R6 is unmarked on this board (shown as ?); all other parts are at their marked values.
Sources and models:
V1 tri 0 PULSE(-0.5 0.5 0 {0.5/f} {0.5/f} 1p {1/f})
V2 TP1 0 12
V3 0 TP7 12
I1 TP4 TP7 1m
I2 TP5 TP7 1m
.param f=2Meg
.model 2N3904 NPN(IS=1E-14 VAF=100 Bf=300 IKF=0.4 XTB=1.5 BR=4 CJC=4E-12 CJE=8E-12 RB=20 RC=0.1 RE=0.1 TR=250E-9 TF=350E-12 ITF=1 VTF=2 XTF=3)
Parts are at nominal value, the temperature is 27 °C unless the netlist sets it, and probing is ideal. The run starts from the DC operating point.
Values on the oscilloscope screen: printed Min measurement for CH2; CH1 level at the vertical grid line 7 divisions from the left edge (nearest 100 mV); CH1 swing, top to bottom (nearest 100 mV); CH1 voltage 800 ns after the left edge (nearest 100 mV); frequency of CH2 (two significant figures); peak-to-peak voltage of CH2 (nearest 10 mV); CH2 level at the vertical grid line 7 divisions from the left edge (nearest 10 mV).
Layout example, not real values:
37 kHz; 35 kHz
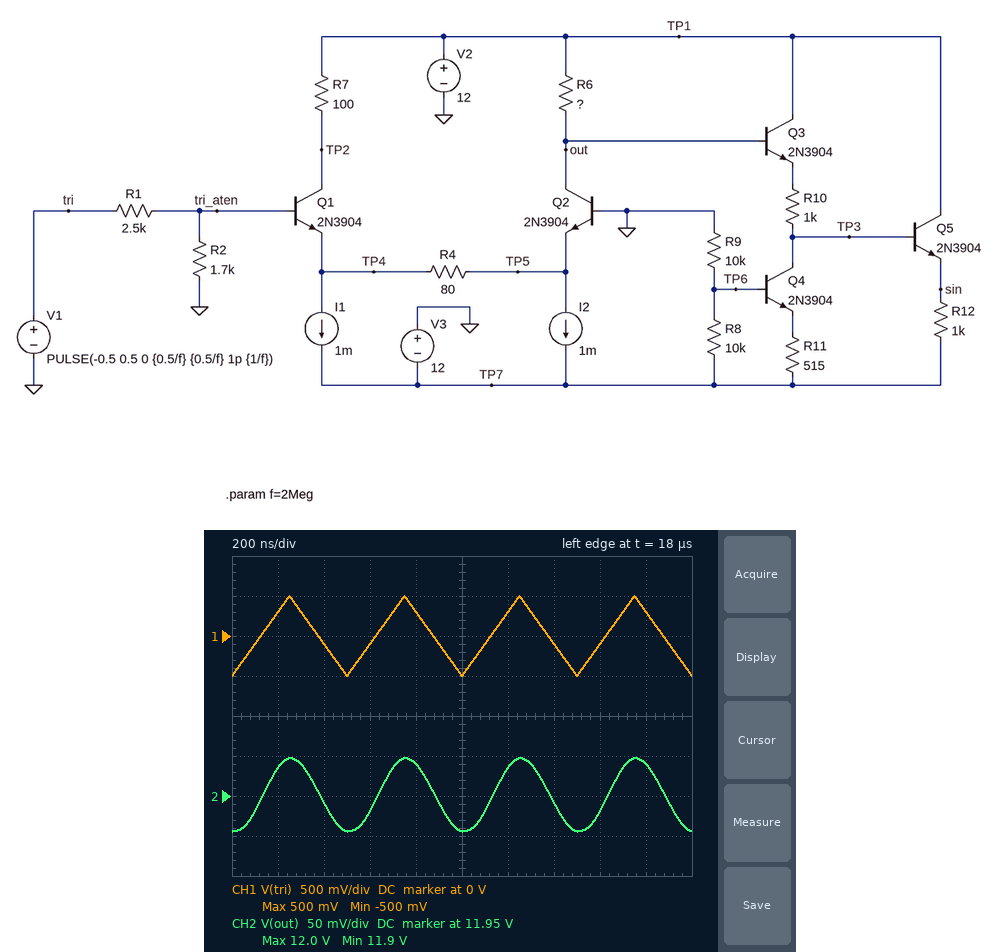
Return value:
11.9 V; -100 mV; 1.0 V; 300 mV; 2.0 MHz; 90 mV; 11.94 V
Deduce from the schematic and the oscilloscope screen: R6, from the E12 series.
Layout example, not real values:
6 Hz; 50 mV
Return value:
47 Ω
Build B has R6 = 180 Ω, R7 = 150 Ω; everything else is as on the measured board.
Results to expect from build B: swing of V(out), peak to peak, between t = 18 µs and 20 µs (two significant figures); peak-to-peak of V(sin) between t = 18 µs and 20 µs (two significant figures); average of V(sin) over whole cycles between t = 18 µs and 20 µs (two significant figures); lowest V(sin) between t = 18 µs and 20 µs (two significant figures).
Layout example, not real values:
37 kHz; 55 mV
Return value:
350 mV; 320 mV; 410 mV; 250 mV
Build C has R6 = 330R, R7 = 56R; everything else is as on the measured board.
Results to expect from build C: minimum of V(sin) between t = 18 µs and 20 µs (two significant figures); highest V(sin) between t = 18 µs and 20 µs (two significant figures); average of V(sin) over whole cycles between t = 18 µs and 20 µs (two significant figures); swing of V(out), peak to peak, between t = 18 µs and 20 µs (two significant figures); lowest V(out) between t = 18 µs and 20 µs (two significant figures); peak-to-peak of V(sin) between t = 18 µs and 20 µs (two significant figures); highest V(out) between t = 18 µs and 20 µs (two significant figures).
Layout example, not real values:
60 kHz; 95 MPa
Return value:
-35 mV; 560 mV; 260 mV; 640 mV; 11 V; 590 mV; 12 V
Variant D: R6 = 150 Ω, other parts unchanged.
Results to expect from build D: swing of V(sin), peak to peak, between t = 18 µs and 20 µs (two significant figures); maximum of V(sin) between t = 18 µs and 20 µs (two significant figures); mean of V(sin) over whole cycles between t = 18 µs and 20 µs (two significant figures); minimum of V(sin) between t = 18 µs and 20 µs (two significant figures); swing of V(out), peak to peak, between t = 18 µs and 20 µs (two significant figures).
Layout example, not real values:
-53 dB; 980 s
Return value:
270 mV; 580 mV; 440 mV; 310 mV; 290 mV
